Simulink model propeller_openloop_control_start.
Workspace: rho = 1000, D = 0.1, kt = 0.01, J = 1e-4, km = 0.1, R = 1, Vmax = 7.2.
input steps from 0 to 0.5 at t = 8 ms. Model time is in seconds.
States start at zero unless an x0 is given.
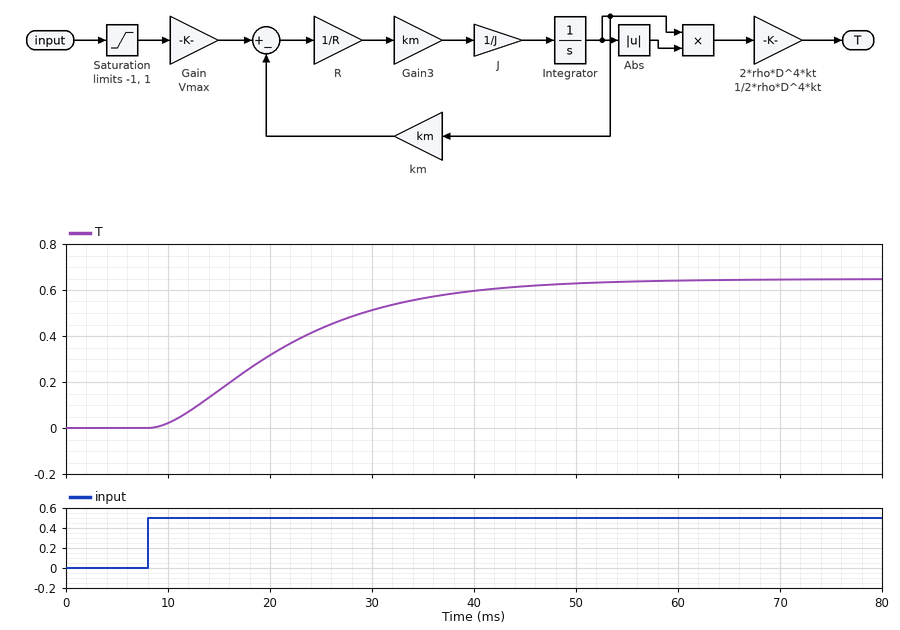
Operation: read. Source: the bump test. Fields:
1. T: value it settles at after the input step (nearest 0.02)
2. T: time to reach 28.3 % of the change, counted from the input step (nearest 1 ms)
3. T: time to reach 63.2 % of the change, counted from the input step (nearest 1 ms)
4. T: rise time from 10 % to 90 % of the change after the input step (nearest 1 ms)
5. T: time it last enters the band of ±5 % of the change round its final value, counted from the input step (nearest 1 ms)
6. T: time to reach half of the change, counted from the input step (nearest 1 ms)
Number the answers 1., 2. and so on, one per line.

1. 0.64
2. 8 ms
3. 16 ms
4. 26 ms
5. 37 ms
6. 12 ms
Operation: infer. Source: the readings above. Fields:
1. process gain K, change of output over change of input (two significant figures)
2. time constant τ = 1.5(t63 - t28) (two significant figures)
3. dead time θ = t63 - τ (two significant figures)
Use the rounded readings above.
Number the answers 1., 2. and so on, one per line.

1. 1.3
2. 12 ms
3. 4.0 ms
